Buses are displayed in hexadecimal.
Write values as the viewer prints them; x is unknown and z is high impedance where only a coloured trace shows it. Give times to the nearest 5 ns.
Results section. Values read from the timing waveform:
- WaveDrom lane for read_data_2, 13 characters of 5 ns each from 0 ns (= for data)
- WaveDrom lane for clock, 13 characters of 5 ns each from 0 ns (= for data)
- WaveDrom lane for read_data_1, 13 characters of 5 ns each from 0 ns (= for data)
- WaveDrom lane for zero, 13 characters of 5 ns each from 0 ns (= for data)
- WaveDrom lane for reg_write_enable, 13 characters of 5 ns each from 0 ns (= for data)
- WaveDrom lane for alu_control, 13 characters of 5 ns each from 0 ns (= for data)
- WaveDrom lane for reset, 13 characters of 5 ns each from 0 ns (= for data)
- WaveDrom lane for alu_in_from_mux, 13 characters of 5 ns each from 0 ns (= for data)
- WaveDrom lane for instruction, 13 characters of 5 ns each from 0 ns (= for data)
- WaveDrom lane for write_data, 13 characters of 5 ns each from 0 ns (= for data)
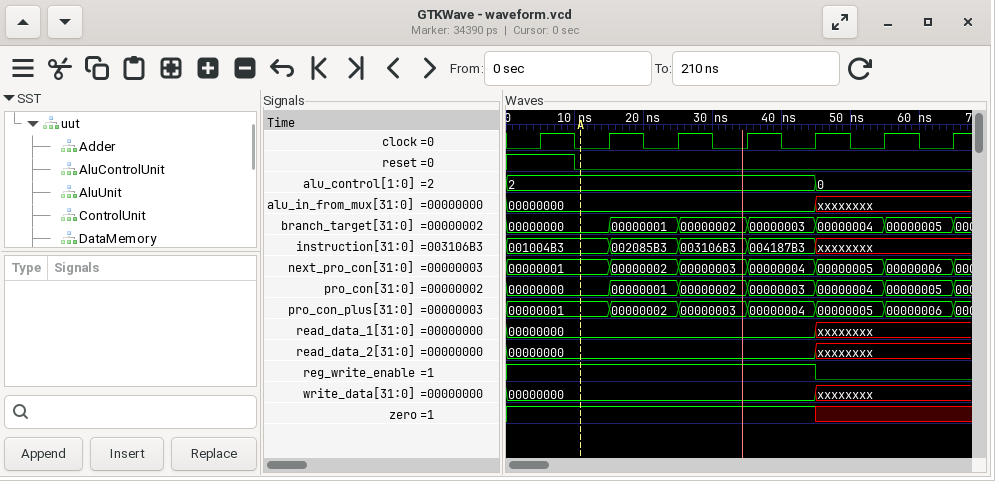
{name: 'read_data_2', wave: '=........x...', data: '00000000'}
{name: 'clock', wave: '0101010101010'}
{name: 'read_data_1', wave: '=........x...', data: '00000000'}
{name: 'zero', wave: '1........x...'}
{name: 'reg_write_enable', wave: '1........0...'}
{name: 'alu_control', wave: '=........=...', data: '2 0'}
{name: 'reset', wave: '1.0..........'}
{name: 'alu_in_from_mux', wave: '=........x...', data: '00000000'}
{name: 'instruction', wave: '=..=.=.=.x...', data: '001004B3 002085B3 003106B3 004187B3'}
{name: 'write_data', wave: '=........x...', data: '00000000'}
